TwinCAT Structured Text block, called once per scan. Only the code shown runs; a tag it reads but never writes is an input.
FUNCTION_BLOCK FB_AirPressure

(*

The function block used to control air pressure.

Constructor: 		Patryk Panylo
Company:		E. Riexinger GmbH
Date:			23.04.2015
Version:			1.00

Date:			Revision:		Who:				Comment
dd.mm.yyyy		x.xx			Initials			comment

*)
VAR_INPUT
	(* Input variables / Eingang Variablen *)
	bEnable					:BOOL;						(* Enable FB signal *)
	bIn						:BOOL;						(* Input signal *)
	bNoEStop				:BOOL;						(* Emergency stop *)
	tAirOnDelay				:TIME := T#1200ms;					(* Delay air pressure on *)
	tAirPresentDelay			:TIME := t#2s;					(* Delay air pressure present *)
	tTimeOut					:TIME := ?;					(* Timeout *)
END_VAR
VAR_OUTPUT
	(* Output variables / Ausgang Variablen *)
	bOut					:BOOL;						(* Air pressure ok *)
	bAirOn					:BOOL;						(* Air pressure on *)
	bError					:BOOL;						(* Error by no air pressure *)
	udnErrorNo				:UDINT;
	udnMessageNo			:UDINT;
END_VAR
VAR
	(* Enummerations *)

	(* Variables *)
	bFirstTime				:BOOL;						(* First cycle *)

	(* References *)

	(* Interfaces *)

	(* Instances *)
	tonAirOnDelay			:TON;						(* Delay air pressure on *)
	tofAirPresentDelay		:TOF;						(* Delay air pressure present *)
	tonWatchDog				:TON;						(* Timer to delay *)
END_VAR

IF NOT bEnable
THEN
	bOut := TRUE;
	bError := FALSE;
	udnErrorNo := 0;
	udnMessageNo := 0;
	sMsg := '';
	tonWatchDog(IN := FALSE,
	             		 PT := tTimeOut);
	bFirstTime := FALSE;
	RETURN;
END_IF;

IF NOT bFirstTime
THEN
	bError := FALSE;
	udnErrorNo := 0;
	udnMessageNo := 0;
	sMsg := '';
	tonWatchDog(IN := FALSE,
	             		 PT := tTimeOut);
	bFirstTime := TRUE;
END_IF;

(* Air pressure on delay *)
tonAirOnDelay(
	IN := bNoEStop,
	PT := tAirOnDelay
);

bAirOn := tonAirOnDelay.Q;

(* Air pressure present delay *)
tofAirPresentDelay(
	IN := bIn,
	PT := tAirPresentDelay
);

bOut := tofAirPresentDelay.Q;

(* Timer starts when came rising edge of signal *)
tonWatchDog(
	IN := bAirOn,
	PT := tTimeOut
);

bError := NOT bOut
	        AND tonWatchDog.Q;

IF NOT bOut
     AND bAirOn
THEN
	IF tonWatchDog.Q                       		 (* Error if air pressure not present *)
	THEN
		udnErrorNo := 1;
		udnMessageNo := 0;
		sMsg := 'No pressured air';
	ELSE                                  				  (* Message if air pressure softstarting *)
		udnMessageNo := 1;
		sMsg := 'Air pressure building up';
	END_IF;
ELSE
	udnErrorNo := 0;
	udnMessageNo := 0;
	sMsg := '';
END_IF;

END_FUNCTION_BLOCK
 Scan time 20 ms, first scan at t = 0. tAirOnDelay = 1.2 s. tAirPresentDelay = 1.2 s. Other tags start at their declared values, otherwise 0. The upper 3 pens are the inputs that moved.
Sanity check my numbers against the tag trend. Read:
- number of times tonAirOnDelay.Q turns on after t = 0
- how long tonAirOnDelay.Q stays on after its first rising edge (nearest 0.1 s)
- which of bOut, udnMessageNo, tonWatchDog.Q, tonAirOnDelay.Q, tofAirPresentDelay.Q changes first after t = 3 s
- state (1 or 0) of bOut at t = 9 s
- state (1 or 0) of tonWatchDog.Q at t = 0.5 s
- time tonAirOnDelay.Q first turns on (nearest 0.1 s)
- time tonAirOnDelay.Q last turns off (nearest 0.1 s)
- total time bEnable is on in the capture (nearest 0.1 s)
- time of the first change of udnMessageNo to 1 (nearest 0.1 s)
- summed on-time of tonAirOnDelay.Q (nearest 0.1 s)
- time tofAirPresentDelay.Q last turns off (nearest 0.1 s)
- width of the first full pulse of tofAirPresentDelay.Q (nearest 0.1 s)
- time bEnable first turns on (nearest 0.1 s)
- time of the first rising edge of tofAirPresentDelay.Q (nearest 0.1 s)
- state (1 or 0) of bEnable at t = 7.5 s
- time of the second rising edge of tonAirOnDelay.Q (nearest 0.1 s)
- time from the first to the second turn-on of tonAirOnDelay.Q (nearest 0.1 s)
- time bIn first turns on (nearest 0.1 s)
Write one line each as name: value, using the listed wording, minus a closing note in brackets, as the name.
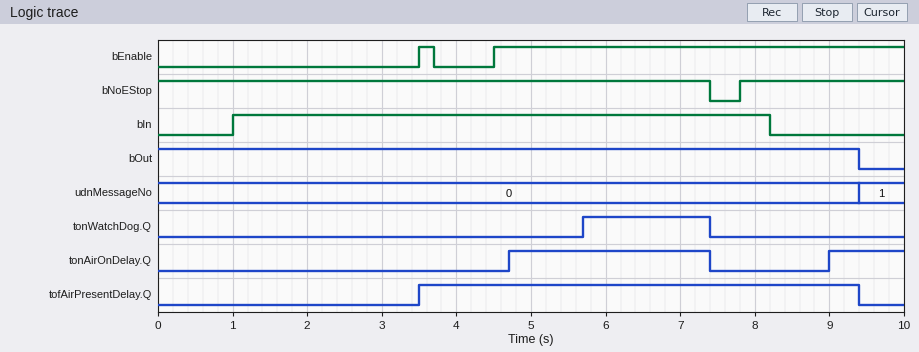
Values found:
number of times tonAirOnDelay.Q turns on after t = 0: 2
how long tonAirOnDelay.Q stays on after its first rising edge: 2.7 s
which of bOut, udnMessageNo, tonWatchDog.Q, tonAirOnDelay.Q, tofAirPresentDelay.Q changes first after t = 3 s: tofAirPresentDelay.Q
state (1 or 0) of bOut at t = 9 s: 1
state (1 or 0) of tonWatchDog.Q at t = 0.5 s: 0
time tonAirOnDelay.Q first turns on: 4.7 s
time tonAirOnDelay.Q last turns off: 7.4 s
total time bEnable is on in the capture: 5.7 s
time of the first change of udnMessageNo to 1: 9.4 s
summed on-time of tonAirOnDelay.Q: 3.7 s
time tofAirPresentDelay.Q last turns off: 9.4 s
width of the first full pulse of tofAirPresentDelay.Q: 5.9 s
time bEnable first turns on: 3.5 s
time of the first rising edge of tofAirPresentDelay.Q: 3.5 s
state (1 or 0) of bEnable at t = 7.5 s: 1
time of the second rising edge of tonAirOnDelay.Q: 9.0 s
time from the first to the second turn-on of tonAirOnDelay.Q: 4.3 s
time bIn first turns on: 1.0 s
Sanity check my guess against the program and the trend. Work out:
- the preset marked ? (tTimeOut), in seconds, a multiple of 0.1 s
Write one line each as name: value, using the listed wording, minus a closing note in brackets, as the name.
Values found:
the preset marked ? (tTimeOut), in seconds, a multiple of 0.1 s: 1.0 s
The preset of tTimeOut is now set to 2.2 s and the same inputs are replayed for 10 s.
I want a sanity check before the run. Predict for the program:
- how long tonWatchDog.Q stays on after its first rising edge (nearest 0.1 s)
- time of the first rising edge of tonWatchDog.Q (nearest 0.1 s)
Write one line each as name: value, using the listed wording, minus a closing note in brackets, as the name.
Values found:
how long tonWatchDog.Q stays on after its first rising edge: 0.5 s
time of the first rising edge of tonWatchDog.Q: 6.9 s
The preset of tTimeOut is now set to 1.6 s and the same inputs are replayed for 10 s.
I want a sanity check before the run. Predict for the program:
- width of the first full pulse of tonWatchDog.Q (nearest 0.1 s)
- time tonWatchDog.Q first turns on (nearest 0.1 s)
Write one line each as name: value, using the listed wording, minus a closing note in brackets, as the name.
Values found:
width of the first full pulse of tonWatchDog.Q: 1.1 s
time tonWatchDog.Q first turns on: 6.3 s
